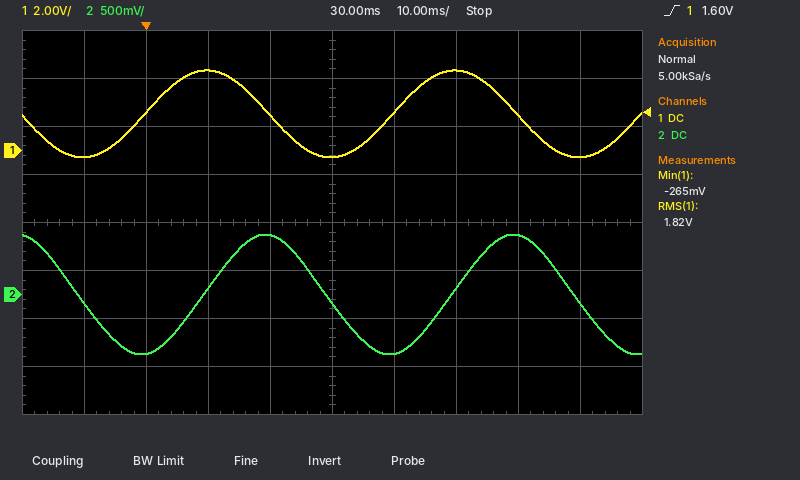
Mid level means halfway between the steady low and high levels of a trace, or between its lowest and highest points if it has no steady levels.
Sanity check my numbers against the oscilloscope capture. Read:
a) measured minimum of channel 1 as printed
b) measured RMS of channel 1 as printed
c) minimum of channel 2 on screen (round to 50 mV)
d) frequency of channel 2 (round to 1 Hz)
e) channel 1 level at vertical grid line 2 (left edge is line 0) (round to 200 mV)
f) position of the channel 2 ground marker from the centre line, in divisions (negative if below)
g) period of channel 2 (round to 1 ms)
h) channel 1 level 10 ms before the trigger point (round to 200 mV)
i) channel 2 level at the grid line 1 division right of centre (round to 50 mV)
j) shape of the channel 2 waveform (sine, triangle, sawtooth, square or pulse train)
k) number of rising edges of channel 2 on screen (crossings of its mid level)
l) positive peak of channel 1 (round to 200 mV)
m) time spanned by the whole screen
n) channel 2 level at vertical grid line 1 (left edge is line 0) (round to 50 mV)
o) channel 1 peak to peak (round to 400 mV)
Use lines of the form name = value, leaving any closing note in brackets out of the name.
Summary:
measured minimum of channel 1 as printed = -265 mV
measured RMS of channel 1 as printed = 1.82 V
minimum of channel 2 on screen = -600 mV
frequency of channel 2 = 25 Hz
channel 1 level at vertical grid line 2 (left edge is line 0) = 1.6 V
position of the channel 2 ground marker from the centre line, in divisions = -1.5 div
period of channel 2 = 40 ms
channel 1 level 10 ms before the trigger point = -200 mV
channel 2 level at the grid line 1 division right of centre = -600 mV
shape of the channel 2 waveform = sine
number of rising edges of channel 2 on screen = 2
positive peak of channel 1 = 3.4 V
time spanned by the whole screen = 100 ms
channel 2 level at vertical grid line 1 (left edge is line 0) = -100 mV
channel 1 peak to peak = 3.6 V
